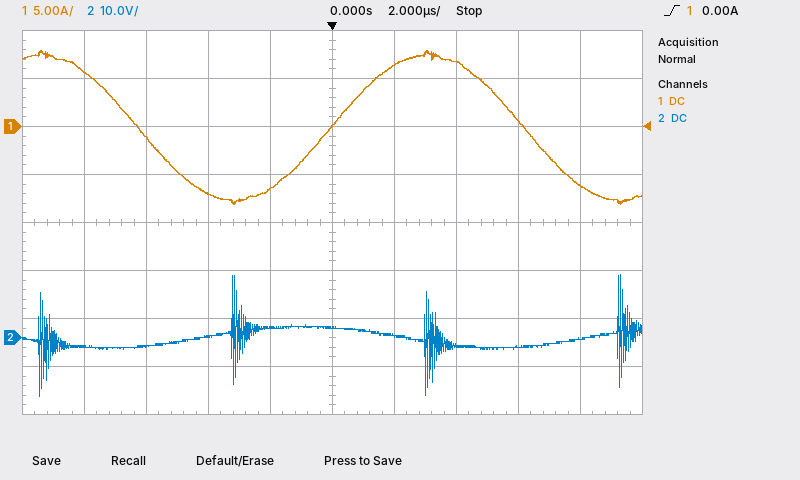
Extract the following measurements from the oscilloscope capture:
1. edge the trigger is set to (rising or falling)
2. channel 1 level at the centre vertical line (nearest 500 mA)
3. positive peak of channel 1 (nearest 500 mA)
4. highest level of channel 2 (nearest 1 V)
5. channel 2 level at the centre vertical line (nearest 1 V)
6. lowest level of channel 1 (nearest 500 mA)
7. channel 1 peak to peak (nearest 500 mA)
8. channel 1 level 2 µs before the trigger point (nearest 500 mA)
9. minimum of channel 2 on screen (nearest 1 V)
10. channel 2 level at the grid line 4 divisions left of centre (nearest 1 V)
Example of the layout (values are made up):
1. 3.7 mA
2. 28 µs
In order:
1. rising
2. 0.0 A
3. 8.0 A
4. 13 V
5. 2 V
6. -8.0 A
7. 16.0 A
8. -6.5 A
9. -12 V
10. -2 V
